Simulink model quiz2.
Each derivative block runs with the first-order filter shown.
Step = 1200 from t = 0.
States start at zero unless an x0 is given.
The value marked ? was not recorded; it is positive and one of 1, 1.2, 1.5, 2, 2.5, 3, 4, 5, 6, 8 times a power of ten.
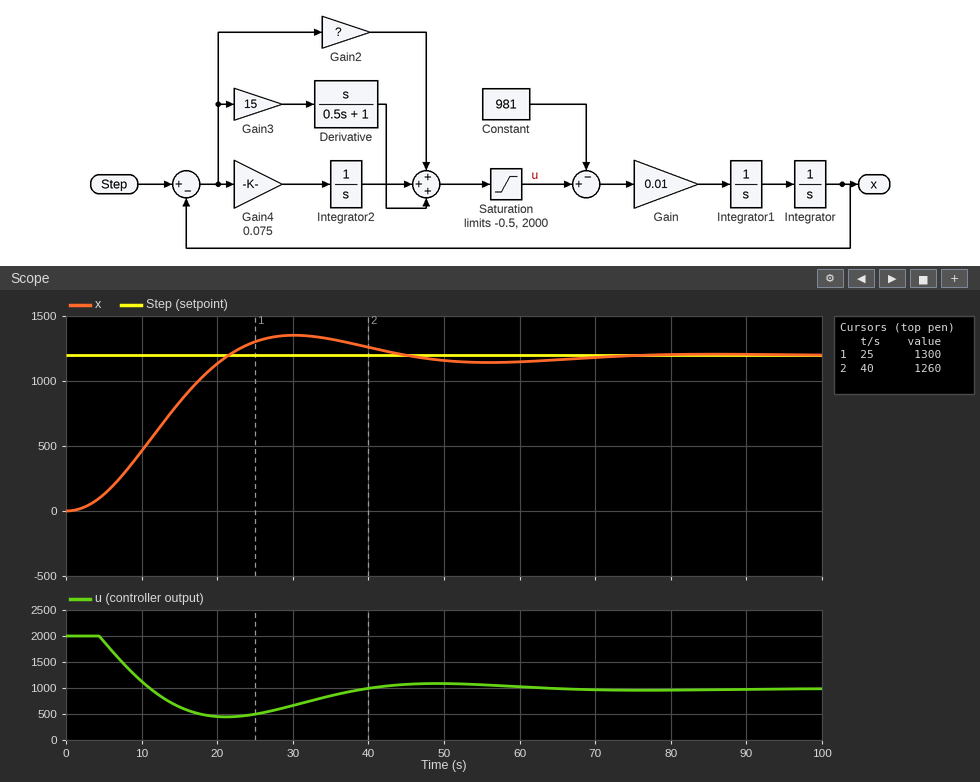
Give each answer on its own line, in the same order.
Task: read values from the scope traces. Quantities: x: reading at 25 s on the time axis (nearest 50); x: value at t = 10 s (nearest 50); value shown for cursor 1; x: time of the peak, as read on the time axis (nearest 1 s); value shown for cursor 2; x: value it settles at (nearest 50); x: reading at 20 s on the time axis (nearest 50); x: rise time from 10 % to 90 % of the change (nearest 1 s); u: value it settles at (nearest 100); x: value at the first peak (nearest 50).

1300
450
1300
30 s
1260
1200
1150
14 s
1000
1350
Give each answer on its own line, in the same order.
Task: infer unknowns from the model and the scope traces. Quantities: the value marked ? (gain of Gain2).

2
